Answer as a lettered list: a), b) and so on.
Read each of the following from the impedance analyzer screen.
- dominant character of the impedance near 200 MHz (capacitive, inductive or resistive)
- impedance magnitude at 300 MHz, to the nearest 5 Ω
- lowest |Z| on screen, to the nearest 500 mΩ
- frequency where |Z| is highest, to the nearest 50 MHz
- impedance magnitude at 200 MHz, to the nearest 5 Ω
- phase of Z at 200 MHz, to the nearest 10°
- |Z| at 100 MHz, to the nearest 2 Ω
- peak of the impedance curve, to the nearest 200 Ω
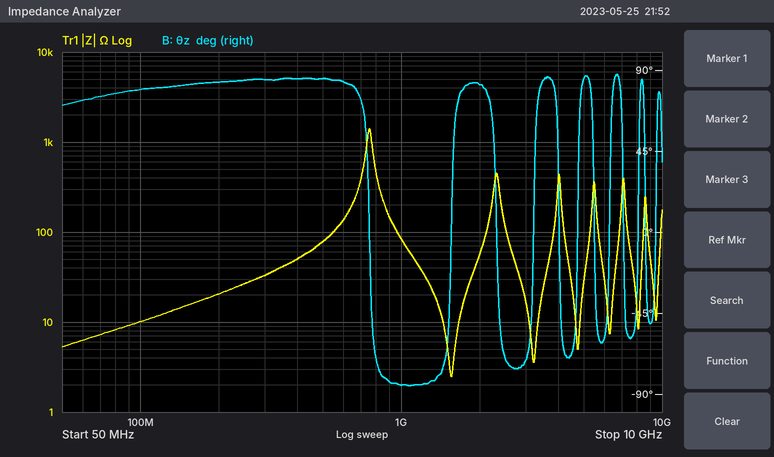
a) inductive
b) 35 Ω
c) 2.5 Ω
d) 750 MHz
e) 20 Ω
f) 80°
g) 10 Ω
h) 1.4 kΩ
